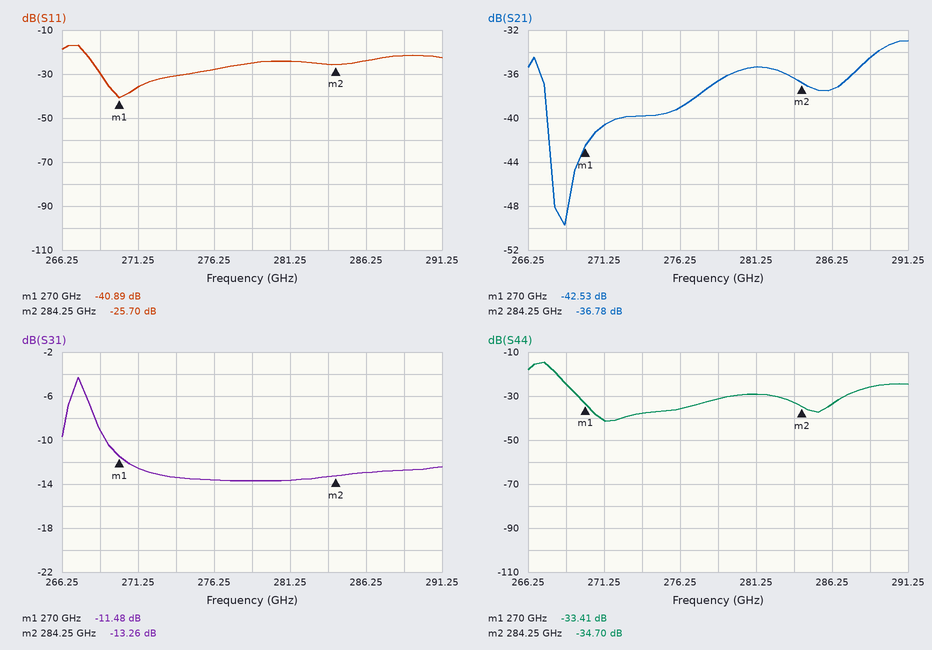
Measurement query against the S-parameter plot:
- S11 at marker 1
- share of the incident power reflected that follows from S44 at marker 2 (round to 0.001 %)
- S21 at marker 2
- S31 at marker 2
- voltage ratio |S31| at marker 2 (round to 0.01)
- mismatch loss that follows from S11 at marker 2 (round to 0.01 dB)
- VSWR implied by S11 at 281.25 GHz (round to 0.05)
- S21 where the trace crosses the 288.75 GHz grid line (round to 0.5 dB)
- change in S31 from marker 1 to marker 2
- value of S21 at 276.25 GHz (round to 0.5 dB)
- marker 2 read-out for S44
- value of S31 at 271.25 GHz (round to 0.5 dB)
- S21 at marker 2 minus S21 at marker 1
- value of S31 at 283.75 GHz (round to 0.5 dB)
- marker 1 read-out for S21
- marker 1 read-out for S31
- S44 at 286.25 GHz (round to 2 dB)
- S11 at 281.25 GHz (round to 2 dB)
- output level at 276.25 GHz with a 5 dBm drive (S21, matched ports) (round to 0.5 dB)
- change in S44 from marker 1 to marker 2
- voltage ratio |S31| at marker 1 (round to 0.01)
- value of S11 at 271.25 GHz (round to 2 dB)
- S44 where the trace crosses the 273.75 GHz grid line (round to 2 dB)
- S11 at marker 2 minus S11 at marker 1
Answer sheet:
-40.89 dB
0.034 %
-36.78 dB
-13.26 dB
0.22
0.01 dB
1.15
-34.5 dB
-1.78 dB
-39.0 dB
-34.70 dB
-12.5 dB
5.75 dB
-13.5 dB
-42.53 dB
-11.48 dB
-34 dB
-24 dB
-34.0 dBm
-1.29 dB
0.27
-36 dB
-38 dB
15.19 dB
